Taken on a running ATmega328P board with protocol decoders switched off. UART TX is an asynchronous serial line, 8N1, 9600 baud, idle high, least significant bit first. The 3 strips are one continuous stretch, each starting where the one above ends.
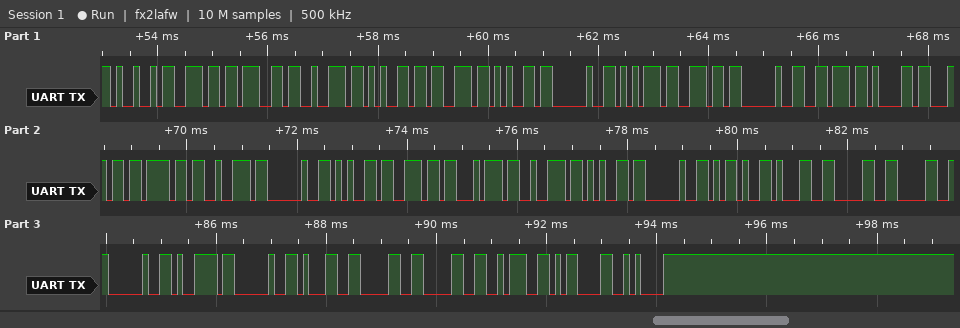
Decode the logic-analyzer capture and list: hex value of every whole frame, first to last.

0x49 0x6E 0x67 0x72 0x65 0x73 0x65 0x20 0x75 0x6E 0x20 0x76 0x61 0x6C 0x6F 0x72 0x20 0x65 0x6E 0x74 0x72 0x65 0x20 0x2D 0x31 0x30 0x30 0x20 0x79 0x20 0x31 0x30 0x30 0x3A 0x0D 0x0A
